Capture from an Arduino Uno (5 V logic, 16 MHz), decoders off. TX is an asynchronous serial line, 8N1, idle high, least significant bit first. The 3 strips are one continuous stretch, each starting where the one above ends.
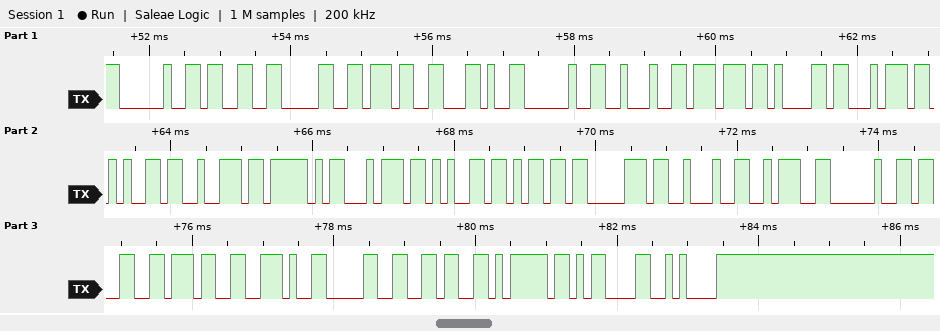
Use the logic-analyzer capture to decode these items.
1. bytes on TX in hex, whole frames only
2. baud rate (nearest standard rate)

20 33 30 37 2C 20 22 77 61 74 65 72 5F 74 65 6D 70 22 3A 20 33 37 2E 30 36 7D 0D 0A
9600 baud
